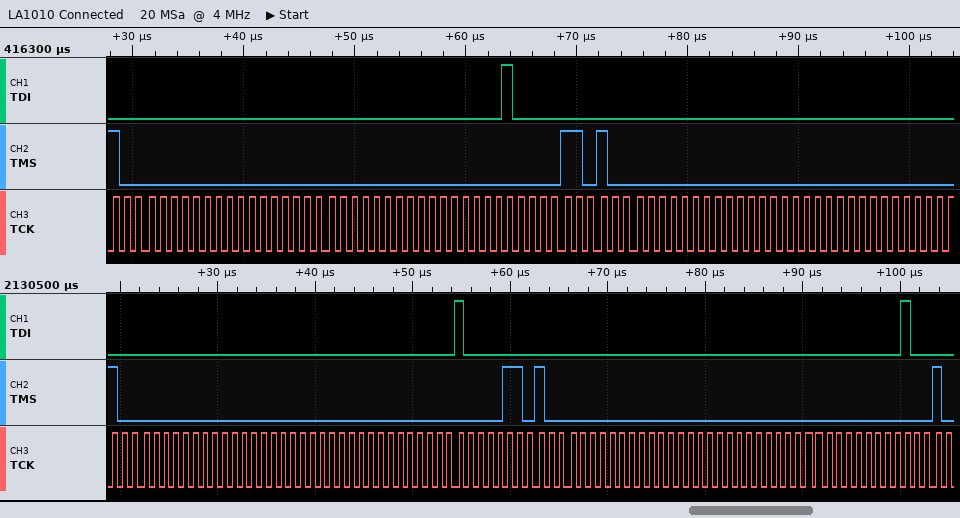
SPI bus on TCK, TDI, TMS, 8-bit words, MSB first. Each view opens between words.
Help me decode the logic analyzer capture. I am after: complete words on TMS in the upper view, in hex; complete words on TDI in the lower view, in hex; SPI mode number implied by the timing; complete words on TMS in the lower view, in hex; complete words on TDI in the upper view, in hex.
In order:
80, 00, 00, 00, 00, D0, 00, 00, 00
00, 00, 00, 00, 10, 00, 00, 00, 00, 00
0
80, 00, 00, 00, 00, D0, 00, 00, 00, 00
00, 00, 00, 00, 10, 00, 00, 00, 00
